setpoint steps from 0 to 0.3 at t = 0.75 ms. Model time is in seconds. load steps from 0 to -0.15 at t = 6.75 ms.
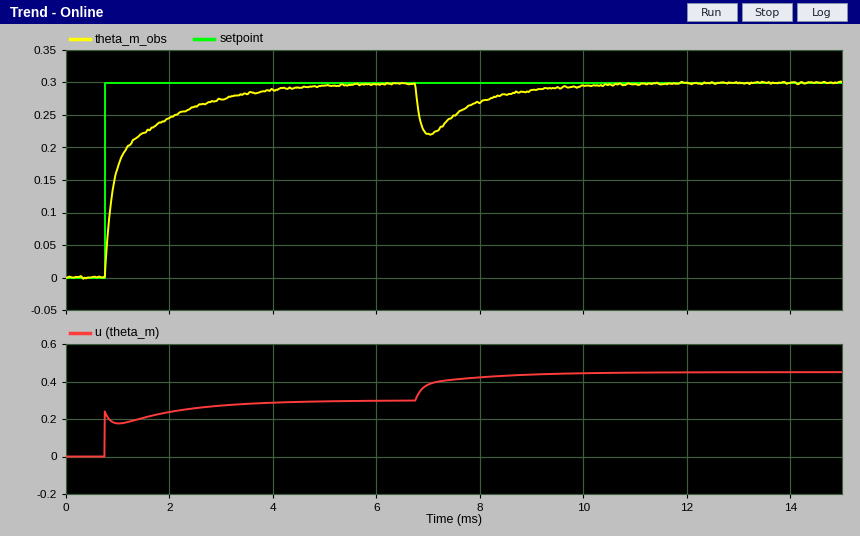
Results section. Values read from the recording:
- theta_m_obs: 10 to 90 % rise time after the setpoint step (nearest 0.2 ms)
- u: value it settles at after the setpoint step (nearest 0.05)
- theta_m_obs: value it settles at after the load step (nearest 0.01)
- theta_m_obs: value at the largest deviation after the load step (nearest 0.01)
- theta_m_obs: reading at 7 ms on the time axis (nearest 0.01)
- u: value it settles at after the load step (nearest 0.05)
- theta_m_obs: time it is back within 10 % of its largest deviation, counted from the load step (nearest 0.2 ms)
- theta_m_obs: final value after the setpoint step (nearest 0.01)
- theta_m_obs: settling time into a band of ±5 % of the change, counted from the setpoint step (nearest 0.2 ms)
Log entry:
2.0 ms
0.30
0.30
0.22
0.22
0.45
2.8 ms
0.30
3.0 ms
